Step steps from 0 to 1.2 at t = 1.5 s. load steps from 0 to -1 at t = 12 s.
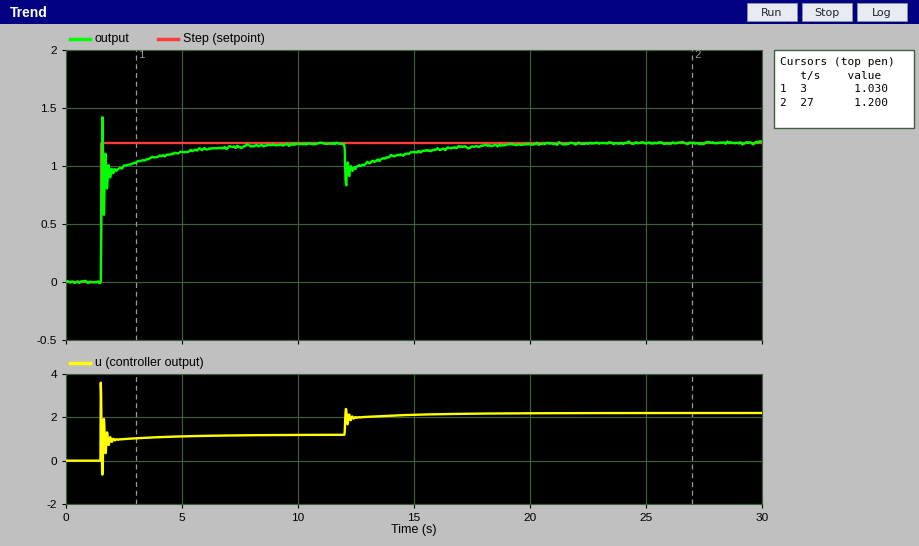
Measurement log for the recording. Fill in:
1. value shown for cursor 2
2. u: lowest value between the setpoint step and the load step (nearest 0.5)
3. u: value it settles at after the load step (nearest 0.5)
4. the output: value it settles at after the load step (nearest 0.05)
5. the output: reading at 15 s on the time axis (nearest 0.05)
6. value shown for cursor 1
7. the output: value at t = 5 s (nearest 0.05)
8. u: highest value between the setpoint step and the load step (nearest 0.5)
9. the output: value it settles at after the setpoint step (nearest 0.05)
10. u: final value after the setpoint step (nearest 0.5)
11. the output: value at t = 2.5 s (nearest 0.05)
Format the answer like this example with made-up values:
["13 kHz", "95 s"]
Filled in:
["1.200", "-0.5", "2.0", "1.20", "1.10", "1.030", "1.10", "3.5", "1.20", "1.0", "1.00"]
